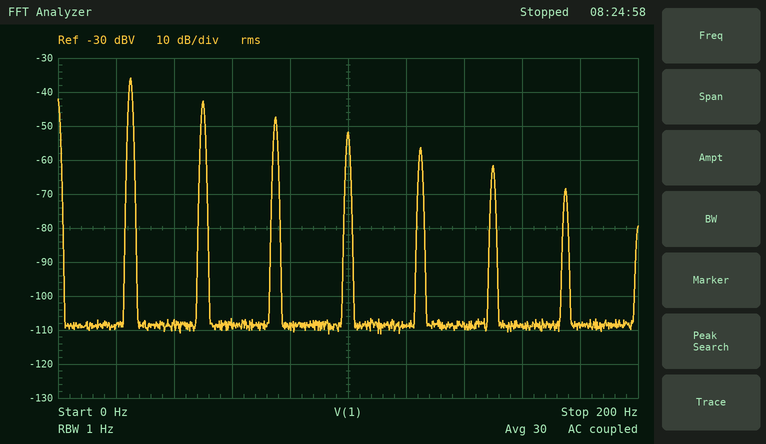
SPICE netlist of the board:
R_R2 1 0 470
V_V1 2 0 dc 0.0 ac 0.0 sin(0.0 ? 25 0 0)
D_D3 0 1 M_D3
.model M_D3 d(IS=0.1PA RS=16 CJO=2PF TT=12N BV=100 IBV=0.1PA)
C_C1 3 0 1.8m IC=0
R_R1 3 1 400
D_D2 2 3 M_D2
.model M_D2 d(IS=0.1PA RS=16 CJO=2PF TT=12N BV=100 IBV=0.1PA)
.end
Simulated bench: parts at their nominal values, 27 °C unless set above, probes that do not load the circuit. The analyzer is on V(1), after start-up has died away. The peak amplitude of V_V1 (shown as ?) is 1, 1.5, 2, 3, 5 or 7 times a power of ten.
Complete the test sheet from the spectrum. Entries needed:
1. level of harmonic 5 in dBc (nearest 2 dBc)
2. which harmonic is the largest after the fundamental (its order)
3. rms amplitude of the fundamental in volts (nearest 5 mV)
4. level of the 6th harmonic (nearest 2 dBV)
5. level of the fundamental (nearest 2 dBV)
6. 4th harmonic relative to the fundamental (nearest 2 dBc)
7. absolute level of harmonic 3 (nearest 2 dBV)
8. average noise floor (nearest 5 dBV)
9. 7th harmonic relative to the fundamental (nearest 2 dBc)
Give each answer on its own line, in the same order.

-20 dBc
2
15 mV
-62 dBV
-36 dBV
-16 dBc
-48 dBV
-110 dBV
-32 dBc
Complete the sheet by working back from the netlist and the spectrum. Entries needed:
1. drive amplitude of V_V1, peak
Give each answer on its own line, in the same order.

7 V
